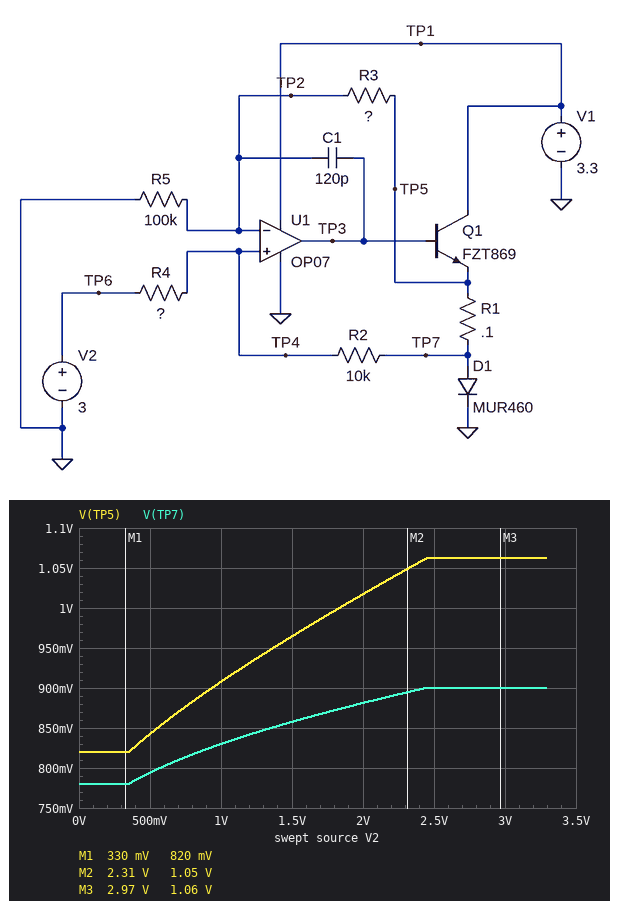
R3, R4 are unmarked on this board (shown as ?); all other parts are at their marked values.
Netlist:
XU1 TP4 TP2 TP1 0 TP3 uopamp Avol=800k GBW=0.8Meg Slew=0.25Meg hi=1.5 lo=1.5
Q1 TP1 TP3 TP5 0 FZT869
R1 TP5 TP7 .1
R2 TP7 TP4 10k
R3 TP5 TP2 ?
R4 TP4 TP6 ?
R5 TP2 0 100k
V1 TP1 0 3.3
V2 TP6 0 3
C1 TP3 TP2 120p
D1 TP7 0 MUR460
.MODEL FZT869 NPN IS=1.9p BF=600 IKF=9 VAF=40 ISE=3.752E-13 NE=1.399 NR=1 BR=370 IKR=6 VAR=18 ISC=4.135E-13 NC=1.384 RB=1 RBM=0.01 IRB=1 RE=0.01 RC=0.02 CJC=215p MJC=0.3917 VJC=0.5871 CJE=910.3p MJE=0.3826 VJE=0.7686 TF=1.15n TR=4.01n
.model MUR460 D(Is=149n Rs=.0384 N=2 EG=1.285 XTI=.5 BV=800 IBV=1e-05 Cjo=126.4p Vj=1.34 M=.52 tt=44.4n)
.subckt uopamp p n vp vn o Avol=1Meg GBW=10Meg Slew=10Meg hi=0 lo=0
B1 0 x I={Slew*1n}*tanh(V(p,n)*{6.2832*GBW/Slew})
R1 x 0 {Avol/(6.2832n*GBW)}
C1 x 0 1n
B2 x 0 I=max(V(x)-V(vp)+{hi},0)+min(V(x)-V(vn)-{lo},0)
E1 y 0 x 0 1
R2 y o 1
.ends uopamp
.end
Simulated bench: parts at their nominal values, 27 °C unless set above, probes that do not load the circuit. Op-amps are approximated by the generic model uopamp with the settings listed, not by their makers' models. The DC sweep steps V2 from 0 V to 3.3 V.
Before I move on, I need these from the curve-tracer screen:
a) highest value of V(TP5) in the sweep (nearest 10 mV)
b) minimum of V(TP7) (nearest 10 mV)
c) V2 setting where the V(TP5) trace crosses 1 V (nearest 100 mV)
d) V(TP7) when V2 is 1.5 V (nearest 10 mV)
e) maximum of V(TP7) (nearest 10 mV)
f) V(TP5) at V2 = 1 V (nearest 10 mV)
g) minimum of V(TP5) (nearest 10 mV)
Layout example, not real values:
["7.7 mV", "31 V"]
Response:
["1.06 V", "780 mV", "1.8 V", "860 mV", "900 mV", "910 mV", "820 mV"]
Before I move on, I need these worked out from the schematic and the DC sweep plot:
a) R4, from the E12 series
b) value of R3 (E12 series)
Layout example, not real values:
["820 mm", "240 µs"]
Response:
["180 kΩ", "8.2 kΩ"]
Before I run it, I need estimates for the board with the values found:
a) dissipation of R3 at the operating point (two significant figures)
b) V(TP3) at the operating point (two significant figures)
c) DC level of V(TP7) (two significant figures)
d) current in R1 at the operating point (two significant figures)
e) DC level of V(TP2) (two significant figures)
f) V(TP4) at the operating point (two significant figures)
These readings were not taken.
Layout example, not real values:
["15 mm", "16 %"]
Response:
["790 nW", "1.8 V", "900 mV", "1.6 A", "980 mV", "1.0 V"]
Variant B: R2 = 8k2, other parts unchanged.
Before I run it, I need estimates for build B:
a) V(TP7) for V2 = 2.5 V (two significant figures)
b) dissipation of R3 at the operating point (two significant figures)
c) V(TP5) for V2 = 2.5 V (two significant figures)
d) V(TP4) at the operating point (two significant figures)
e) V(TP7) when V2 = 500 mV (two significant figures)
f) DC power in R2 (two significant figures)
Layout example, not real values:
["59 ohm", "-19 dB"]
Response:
["890 mV", "790 nW", "1.0 V", "990 mV", "800 mV", "1.0 µW"]
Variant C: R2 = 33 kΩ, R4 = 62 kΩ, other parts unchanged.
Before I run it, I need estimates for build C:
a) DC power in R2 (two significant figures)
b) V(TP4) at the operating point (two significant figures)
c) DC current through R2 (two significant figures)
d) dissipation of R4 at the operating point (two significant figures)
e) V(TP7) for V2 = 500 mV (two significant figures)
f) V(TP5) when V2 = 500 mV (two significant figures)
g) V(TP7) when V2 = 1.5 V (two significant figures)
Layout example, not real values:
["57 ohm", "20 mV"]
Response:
["16 µW", "1.6 V", "22 µA", "30 µW", "780 mV", "820 mV", "900 mV"]
